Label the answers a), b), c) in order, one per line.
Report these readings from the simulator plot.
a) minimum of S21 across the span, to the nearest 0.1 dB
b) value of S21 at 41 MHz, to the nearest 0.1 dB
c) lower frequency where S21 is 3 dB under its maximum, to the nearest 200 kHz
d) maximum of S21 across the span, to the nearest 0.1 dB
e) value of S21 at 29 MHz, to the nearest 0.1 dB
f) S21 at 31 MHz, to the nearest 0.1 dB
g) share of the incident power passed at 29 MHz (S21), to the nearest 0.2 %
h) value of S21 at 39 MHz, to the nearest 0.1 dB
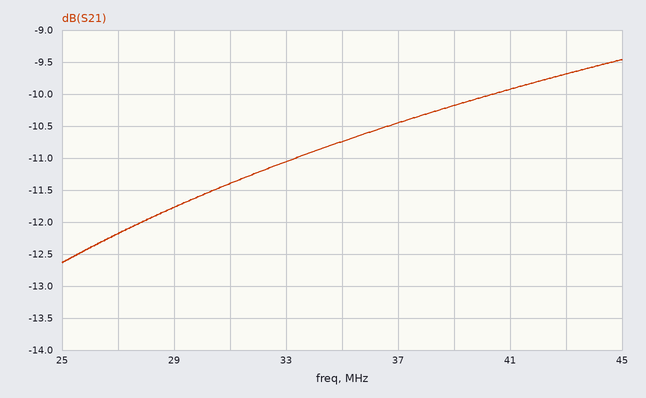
a) -12.6 dB
b) -9.9 dB
c) 25.8 MHz
d) -9.5 dB
e) -11.8 dB
f) -11.4 dB
g) 6.6 %
h) -10.2 dB
